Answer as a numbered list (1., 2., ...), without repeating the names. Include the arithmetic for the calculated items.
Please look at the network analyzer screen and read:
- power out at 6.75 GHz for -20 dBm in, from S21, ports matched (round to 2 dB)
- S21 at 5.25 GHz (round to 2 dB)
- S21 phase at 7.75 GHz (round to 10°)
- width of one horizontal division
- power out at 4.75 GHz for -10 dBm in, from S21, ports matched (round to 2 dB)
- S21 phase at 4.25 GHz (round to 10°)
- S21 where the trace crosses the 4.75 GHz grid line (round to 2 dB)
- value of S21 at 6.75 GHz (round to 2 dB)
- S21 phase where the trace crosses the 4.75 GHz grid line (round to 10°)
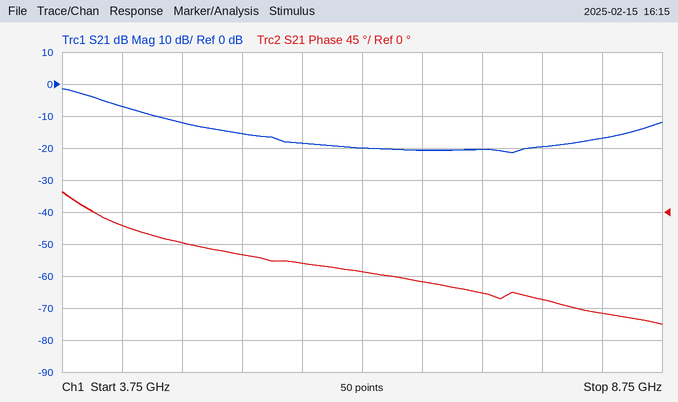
1. -20 dBm + (-20 dB) = -40 dBm
2. -16 dB
3. -120°
4. 500 MHz
5. -10 dBm + (-12 dB) = -22 dBm
6. -20°
7. -12 dB
8. -20 dB
9. -40°
